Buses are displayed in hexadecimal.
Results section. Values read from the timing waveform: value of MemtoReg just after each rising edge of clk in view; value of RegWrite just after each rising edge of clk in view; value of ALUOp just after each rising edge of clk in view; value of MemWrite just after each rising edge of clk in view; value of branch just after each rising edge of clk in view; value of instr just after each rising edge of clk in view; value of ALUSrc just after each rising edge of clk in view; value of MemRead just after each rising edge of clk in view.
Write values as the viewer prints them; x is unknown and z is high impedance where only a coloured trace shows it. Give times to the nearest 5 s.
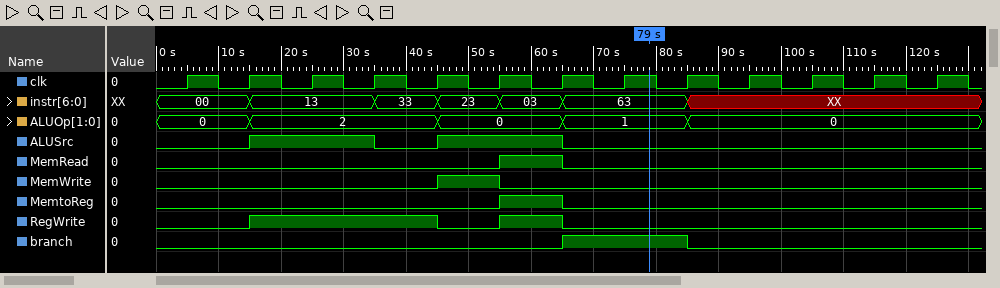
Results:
0 0 0 0 0 1 0 0 0 0 0 0 0
0 1 1 1 0 1 0 0 0 0 0 0 0
0, 2, 2, 2, 0, 0, 1, 1, 0, 0, 0, 0, 0
0 0 0 0 1 0 0 0 0 0 0 0 0
0 0 0 0 0 0 1 1 0 0 0 0 0
00, 13, 13, 33, 23, 03, 63, 63, XX, XX, XX, XX, XX
0 1 1 0 1 1 0 0 0 0 0 0 0
0 0 0 0 0 1 0 0 0 0 0 0 0
